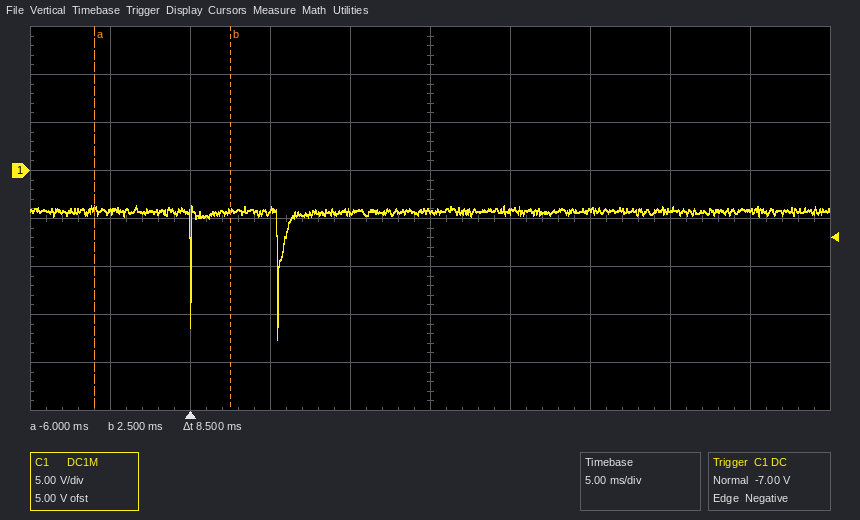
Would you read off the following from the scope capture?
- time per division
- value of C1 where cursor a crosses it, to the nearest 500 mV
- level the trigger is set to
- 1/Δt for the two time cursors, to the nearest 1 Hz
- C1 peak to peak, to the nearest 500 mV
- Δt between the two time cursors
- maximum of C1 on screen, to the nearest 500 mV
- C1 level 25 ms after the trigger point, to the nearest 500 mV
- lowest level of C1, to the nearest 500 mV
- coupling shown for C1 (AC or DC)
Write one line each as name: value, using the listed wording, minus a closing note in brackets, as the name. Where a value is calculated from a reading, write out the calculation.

time per division: 5 ms
value of C1 where cursor a crosses it, to the nearest 500 mV: -4.0 V
level the trigger is set to: -7.00 V
1/Δt for the two time cursors, to the nearest 1 Hz: 1 / 8.5 ms ≈ 118 Hz
C1 peak to peak, to the nearest 500 mV: -3.5 V − (-17.5 V) = 14.0 V
Δt between the two time cursors: 8.5 ms
maximum of C1 on screen, to the nearest 500 mV: -3.5 V
C1 level 25 ms after the trigger point, to the nearest 500 mV: -4.0 V
lowest level of C1, to the nearest 500 mV: -17.5 V
coupling shown for C1: DC
